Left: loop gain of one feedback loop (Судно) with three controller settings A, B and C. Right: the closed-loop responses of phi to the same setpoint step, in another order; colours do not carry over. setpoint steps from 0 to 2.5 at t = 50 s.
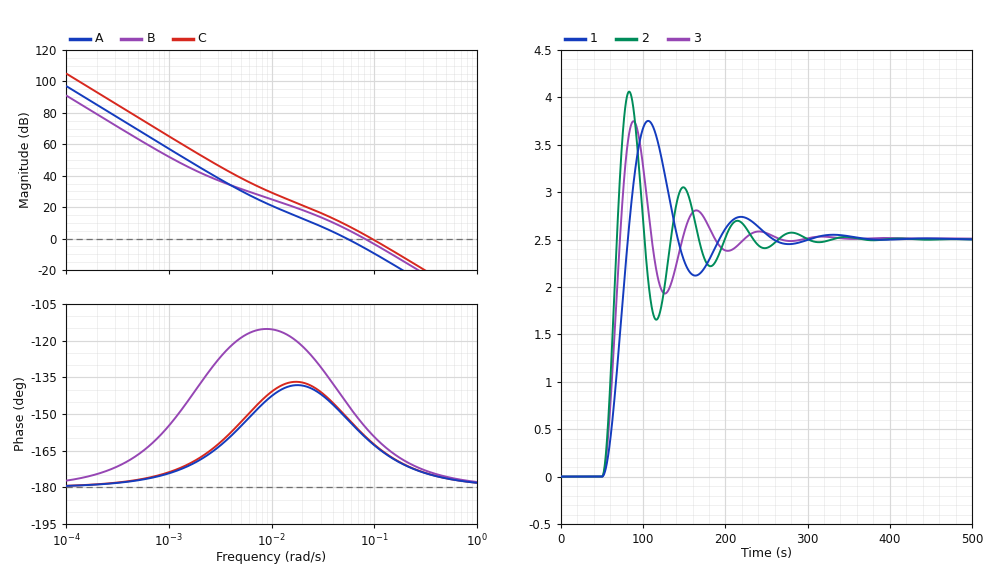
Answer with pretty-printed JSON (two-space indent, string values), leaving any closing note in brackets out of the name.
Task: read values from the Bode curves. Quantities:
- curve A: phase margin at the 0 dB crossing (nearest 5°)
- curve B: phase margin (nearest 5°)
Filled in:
{
  "curve A: phase margin at the 0 dB crossing": "30°",
  "curve B: phase margin": "25°"
}
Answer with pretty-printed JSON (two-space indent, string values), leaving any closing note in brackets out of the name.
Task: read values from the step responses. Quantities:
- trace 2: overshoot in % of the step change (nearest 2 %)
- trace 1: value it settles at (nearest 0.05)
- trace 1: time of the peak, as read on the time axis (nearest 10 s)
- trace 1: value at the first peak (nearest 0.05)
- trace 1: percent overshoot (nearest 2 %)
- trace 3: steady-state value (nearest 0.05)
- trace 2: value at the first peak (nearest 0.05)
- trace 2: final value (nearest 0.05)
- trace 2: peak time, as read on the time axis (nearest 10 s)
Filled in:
{
  "trace 2: overshoot in % of the step change": "62 %",
  "trace 1: value it settles at": "2.50",
  "trace 1: time of the peak, as read on the time axis": "110 s",
  "trace 1: value at the first peak": "3.75",
  "trace 1: percent overshoot": "50 %",
  "trace 3: steady-state value": "2.50",
  "trace 2: value at the first peak": "4.05",
  "trace 2: final value": "2.50",
  "trace 2: peak time, as read on the time axis": "80 s"
}
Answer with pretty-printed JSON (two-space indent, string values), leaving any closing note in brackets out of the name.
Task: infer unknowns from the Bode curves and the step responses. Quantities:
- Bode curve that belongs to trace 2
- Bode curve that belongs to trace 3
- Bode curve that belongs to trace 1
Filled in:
{
  "Bode curve that belongs to trace 2": "C",
  "Bode curve that belongs to trace 3": "B",
  "Bode curve that belongs to trace 1": "A"
}
